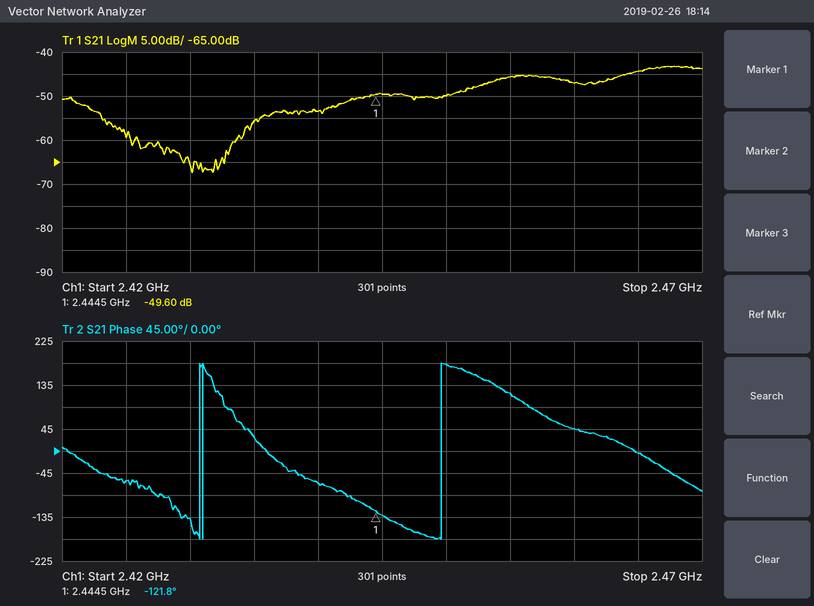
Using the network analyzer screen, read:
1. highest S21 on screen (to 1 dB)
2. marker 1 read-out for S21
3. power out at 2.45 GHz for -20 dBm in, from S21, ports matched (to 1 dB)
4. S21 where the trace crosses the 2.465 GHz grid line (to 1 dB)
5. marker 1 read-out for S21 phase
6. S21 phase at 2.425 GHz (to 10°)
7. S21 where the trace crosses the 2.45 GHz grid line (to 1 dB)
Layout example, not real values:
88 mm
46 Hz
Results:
-43 dB
-49.60 dB
-70 dBm
-44 dB
-121.8°
-60°
-50 dB
